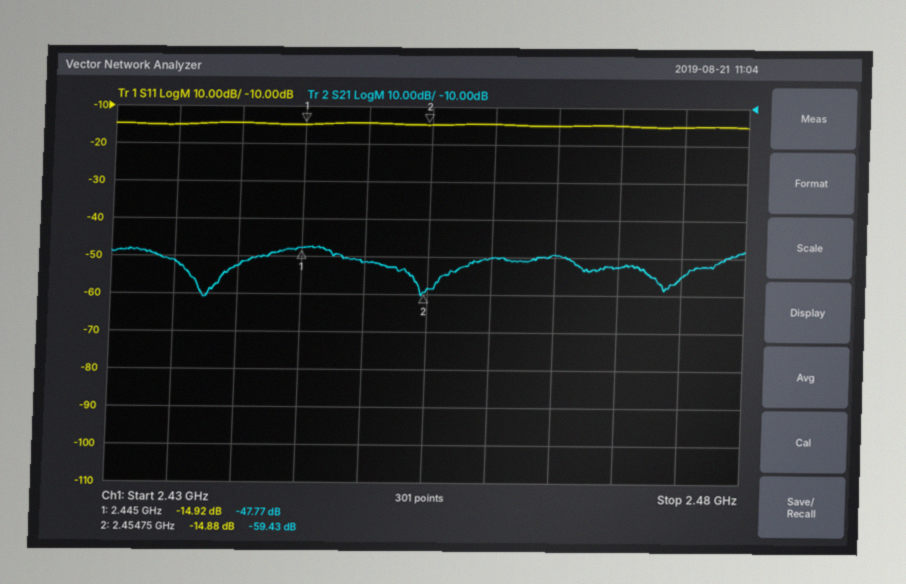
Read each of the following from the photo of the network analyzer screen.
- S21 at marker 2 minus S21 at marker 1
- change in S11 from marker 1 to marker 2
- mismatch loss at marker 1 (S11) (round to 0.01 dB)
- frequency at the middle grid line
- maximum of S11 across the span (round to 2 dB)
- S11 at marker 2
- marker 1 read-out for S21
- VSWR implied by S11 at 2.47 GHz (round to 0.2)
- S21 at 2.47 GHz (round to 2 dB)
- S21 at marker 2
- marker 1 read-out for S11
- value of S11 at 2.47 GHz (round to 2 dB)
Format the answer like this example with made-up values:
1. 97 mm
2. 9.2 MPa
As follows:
1. -11.66 dB
2. 0.04 dB
3. 0.14 dB
4. 2.455 GHz
5. -14 dB
6. -14.88 dB
7. -47.77 dB
8. 1.4
9. -52 dB
10. -59.43 dB
11. -14.92 dB
12. -14 dB
